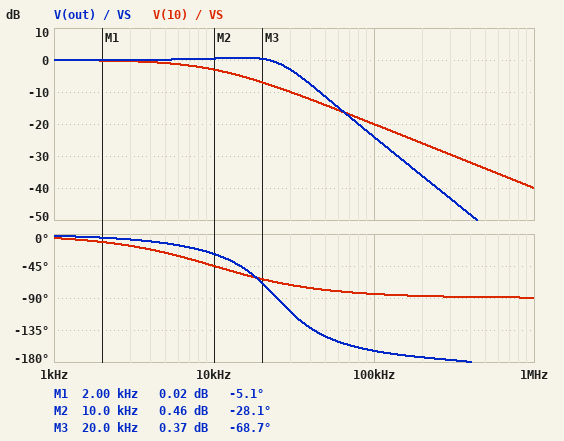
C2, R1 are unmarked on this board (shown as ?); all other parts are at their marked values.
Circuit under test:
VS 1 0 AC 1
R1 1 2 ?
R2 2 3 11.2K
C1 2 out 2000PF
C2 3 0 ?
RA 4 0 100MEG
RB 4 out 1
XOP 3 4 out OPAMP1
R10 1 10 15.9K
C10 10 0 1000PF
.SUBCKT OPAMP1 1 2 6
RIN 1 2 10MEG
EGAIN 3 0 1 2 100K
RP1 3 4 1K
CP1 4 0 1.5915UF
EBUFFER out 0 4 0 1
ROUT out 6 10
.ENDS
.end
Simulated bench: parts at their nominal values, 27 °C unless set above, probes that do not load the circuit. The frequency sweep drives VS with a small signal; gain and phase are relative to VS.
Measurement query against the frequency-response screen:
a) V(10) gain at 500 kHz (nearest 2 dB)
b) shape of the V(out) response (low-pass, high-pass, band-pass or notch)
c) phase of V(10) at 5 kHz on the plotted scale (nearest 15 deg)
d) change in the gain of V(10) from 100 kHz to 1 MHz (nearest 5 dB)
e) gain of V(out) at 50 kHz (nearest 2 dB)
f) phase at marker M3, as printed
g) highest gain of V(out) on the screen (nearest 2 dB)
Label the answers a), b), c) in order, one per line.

a) -34 dB
b) low-pass
c) -30 deg
d) -20 dB
e) -12 dB
f) -68.7 deg
g) 0 dB
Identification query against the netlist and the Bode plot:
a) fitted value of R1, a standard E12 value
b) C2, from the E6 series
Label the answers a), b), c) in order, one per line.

a) 3.9 kΩ
b) 470 pF
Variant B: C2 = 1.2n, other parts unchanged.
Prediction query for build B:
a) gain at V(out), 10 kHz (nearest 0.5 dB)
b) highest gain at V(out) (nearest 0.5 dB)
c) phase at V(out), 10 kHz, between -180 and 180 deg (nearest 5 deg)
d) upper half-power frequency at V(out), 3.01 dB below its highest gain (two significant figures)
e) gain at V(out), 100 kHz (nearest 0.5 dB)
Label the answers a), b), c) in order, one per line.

a) -2.0 dB
b) 0 dB
c) -65 deg
d) 12 kHz
e) -32.5 dB
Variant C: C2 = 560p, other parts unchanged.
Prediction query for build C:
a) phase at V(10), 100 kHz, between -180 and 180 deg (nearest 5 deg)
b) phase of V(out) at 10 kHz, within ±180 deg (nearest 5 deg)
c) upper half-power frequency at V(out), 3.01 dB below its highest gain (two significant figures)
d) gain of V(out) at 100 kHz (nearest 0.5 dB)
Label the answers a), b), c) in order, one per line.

a) -85 deg
b) -35 deg
c) 25 kHz
d) -25.5 dB
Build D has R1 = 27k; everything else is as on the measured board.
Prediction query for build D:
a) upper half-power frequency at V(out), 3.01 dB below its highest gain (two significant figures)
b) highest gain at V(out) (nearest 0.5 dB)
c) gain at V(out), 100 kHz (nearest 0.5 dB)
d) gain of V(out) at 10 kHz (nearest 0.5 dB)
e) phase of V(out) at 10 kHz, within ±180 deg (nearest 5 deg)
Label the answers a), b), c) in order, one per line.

a) 11 kHz
b) 1.0 dB
c) -41.0 dB
d) -1.0 dB
e) -95 deg
